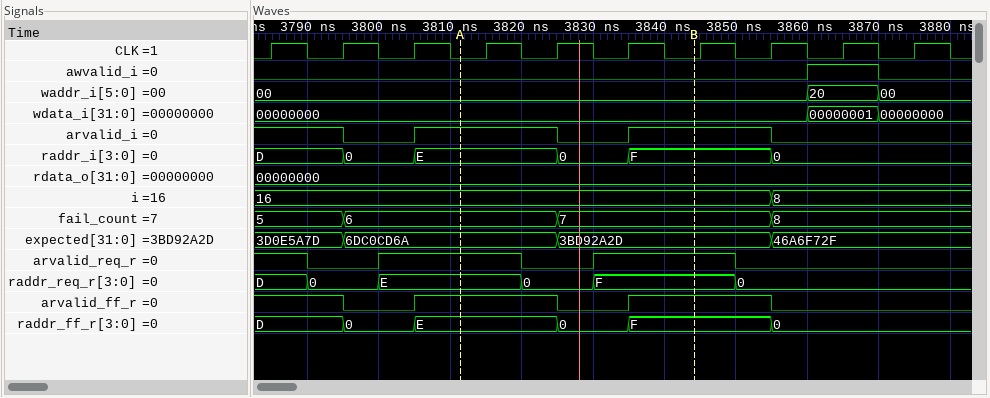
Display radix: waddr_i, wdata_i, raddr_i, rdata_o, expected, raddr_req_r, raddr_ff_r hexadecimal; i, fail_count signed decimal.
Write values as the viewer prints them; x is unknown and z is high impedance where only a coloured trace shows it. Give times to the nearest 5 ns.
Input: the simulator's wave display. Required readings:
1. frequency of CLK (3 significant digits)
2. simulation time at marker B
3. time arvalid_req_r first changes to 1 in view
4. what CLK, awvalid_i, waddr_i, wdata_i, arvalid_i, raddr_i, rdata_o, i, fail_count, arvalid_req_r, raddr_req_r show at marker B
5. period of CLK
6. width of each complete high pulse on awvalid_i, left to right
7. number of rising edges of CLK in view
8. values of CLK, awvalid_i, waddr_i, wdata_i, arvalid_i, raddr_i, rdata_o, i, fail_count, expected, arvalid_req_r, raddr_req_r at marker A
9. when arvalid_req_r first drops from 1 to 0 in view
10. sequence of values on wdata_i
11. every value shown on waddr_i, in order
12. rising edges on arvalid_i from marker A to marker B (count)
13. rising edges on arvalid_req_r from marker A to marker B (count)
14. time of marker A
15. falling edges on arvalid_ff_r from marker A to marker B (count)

100 MHz
3845 ns
3800 ns
CLK=0, awvalid_i=0, waddr_i=00, wdata_i=00000000, arvalid_i=1, raddr_i=F, rdata_o=00000000, i=16, fail_count=7, arvalid_req_r=1, raddr_req_r=F
10 ns
10 ns
10
CLK=0, awvalid_i=0, waddr_i=00, wdata_i=00000000, arvalid_i=1, raddr_i=E, rdata_o=00000000, i=16, fail_count=6, expected=6DC0CD6A, arvalid_req_r=1, raddr_req_r=E
3790 ns
00000000, 00000001, 00000000
00, 20, 00
1
1
3810 ns
1
